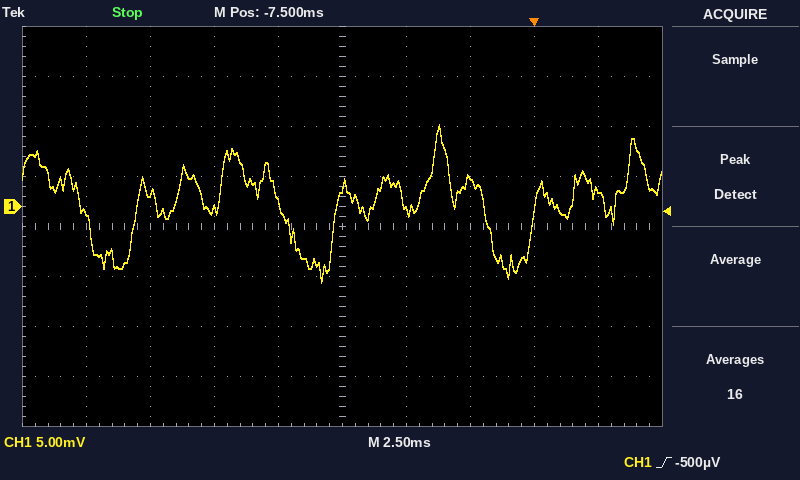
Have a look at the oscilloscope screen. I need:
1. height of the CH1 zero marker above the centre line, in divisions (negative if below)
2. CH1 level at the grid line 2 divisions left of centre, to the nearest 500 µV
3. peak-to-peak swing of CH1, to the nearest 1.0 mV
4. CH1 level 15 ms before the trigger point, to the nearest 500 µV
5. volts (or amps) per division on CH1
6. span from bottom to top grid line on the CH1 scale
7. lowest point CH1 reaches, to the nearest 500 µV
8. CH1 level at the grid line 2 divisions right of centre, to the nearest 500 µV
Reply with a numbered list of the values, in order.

1. +0.4 div
2. -500 µV
3. 16.0 mV
4. 1.5 mV
5. 5 mV
6. 40 mV
7. -7.5 mV
8. 3.0 mV
